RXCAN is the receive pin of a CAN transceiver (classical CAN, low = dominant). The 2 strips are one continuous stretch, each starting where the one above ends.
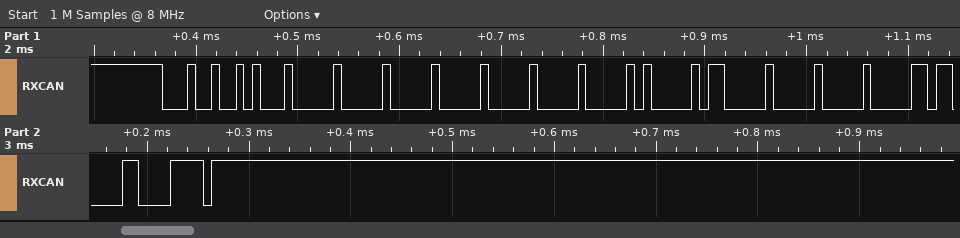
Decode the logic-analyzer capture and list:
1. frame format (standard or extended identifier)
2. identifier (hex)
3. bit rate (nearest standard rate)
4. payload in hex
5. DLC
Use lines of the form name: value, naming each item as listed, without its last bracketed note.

frame format: standard
identifier: 0x125
bit rate: 125 kbit/s
payload in hex: 00 00 00 00 40 C0 00 02
DLC: 8
